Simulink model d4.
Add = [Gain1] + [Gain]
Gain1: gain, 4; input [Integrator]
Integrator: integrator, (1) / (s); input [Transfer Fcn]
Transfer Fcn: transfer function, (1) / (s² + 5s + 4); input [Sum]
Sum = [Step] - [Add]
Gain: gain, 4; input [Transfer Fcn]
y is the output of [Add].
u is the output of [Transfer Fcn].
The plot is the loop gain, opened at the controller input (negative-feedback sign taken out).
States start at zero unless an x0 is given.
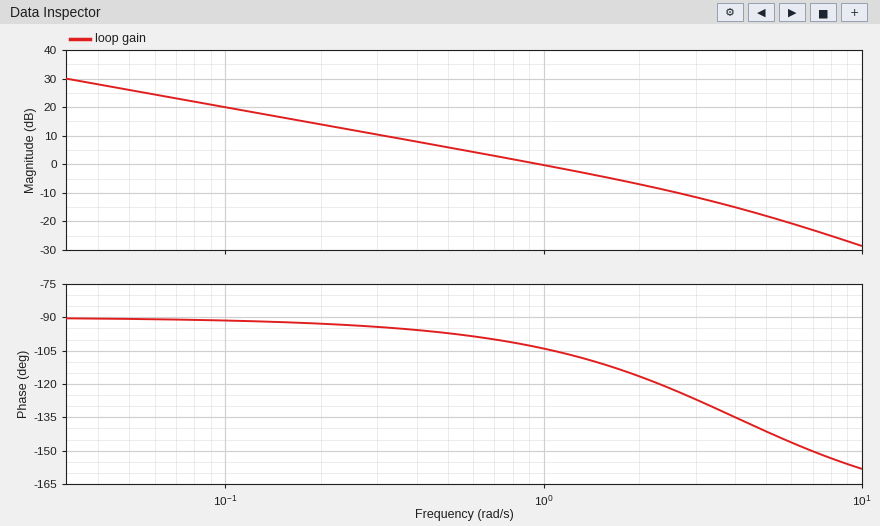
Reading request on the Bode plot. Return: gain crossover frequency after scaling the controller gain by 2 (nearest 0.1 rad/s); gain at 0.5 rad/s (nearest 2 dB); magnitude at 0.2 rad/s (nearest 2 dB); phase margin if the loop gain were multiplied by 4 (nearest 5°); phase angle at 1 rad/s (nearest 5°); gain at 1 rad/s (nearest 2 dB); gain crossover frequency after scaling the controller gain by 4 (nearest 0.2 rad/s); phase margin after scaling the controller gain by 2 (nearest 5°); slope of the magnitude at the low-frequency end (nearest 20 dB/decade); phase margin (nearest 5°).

1.8 rad/s
6 dB
14 dB
50°
-105°
0 dB
3.2 rad/s
65°
-20 dB/decade
75°
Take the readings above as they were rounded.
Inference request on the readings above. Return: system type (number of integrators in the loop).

1
